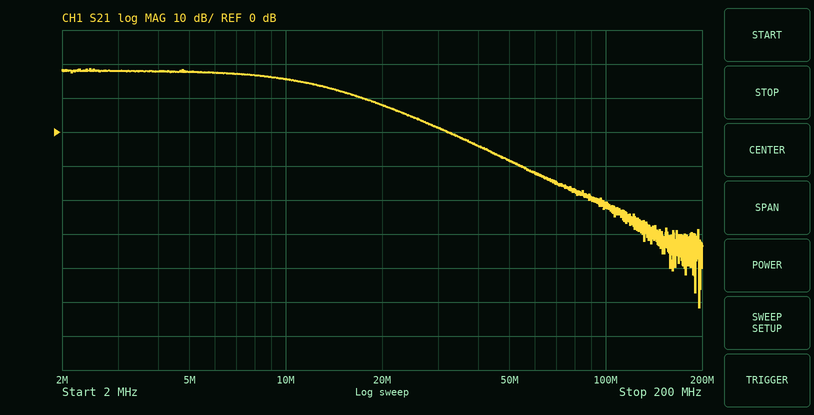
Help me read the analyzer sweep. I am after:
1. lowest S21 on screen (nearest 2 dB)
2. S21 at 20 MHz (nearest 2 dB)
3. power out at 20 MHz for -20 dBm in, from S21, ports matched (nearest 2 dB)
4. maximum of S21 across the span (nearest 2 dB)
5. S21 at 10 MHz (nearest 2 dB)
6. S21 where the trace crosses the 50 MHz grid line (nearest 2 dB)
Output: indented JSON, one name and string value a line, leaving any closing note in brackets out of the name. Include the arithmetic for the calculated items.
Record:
{
  "lowest S21 on screen": "-52 dB",
  "S21 at 20 MHz": "8 dB",
  "power out at 20 MHz for -20 dBm in, from S21, ports matched": "-20 dBm + (8 dB) = -12 dBm",
  "maximum of S21 across the span": "18 dB",
  "S21 at 10 MHz": "16 dB",
  "S21 where the trace crosses the 50 MHz grid line": "-8 dB"
}
